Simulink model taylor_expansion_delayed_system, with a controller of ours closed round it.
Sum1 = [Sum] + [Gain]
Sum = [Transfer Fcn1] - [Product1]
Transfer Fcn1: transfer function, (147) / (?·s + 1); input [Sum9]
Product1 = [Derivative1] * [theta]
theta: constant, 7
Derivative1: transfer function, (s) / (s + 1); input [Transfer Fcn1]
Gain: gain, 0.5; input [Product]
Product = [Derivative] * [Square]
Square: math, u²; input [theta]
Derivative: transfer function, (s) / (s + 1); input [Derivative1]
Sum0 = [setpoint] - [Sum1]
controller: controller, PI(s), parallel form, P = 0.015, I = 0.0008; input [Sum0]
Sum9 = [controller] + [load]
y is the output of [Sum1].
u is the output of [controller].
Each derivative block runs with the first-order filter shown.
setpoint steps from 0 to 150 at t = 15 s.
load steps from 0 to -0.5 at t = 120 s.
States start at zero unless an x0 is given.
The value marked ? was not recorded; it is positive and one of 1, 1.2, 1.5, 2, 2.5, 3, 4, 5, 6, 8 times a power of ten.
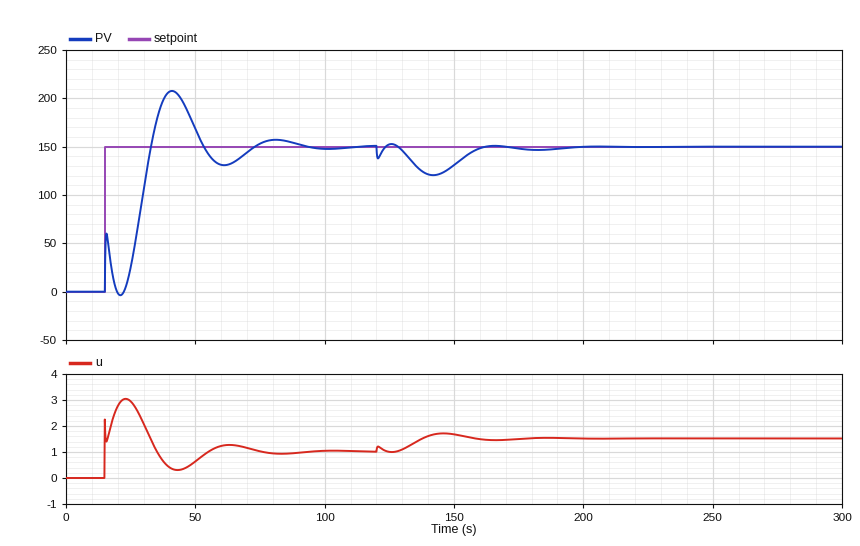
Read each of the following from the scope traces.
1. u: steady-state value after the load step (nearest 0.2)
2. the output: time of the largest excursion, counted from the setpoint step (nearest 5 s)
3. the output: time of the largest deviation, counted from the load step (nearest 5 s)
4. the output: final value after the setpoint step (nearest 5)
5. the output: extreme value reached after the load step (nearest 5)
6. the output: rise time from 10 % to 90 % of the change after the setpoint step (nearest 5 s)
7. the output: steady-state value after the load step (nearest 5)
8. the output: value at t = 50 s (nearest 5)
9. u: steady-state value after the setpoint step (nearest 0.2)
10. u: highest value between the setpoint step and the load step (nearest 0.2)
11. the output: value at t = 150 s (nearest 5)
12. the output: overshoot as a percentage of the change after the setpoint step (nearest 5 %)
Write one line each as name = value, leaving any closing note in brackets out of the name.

u: steady-state value after the load step = 1.6
the output: time of the largest excursion, counted from the setpoint step = 25 s
the output: time of the largest deviation, counted from the load step = 20 s
the output: final value after the setpoint step = 150
the output: extreme value reached after the load step = 120
the output: rise time from 10 % to 90 % of the change after the setpoint step = 15 s
the output: steady-state value after the load step = 150
the output: value at t = 50 s = 170
u: steady-state value after the setpoint step = 1.0
u: highest value between the setpoint step and the load step = 3.0
the output: value at t = 150 s = 130
the output: overshoot as a percentage of the change after the setpoint step = 40 %
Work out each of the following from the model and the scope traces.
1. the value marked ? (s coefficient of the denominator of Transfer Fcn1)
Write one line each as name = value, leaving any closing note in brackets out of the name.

the value marked ? = 20
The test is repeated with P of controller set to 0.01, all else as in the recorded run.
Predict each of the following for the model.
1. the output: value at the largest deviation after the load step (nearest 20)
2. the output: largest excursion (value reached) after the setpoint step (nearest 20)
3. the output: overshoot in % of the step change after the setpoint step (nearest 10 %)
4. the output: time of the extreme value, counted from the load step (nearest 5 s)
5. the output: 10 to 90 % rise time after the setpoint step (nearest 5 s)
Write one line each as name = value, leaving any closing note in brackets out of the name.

the output: value at the largest deviation after the load step = 120
the output: largest excursion (value reached) after the setpoint step = 200
the output: overshoot in % of the step change after the setpoint step = 30 %
the output: time of the extreme value, counted from the load step = 25 s
the output: 10 to 90 % rise time after the setpoint step = 20 s
